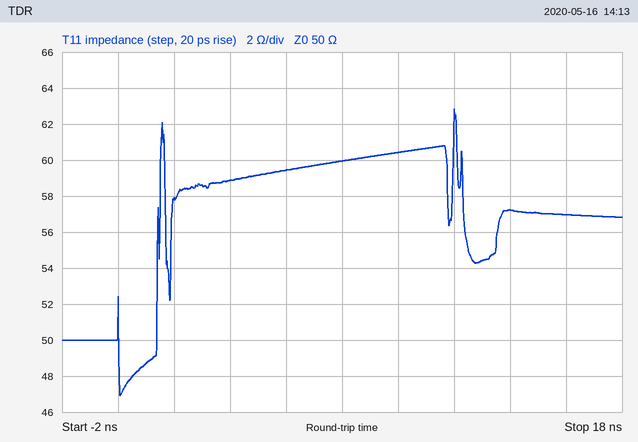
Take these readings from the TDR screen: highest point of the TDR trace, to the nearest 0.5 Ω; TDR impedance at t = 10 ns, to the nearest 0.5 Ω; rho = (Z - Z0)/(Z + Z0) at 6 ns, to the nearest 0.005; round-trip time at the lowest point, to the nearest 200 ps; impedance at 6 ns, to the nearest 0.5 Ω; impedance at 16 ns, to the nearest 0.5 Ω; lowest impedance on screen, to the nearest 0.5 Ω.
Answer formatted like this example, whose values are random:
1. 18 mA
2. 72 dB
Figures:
1. 63.0 Ω
2. 60.5 Ω
3. +0.085
4. 0.0 ns
5. 59.5 Ω
6. 57.0 Ω
7. 47.0 Ω
